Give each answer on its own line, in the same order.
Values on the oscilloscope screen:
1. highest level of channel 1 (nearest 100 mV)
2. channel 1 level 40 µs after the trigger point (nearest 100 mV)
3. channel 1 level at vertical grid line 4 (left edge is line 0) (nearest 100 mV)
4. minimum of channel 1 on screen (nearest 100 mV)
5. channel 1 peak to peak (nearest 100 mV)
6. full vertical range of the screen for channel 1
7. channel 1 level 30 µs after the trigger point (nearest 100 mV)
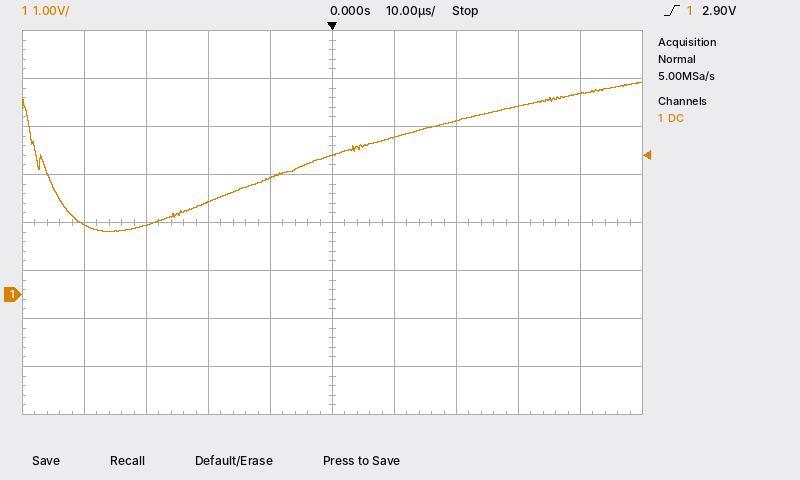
4.4 V
4.2 V
2.4 V
1.3 V
3.1 V
8 V
3.9 V
